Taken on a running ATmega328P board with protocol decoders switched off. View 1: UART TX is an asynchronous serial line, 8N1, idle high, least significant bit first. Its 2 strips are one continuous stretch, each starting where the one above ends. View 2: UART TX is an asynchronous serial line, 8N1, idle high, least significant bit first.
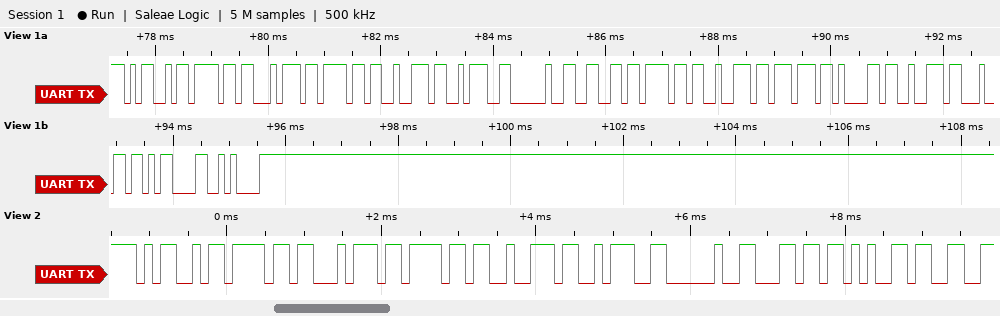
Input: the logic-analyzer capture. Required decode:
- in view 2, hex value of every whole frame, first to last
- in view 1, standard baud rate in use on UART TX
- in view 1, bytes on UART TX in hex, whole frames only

0x4D 0x6F 0x74 0x6F 0x72 0x3A 0x20 0x6C 0x65
9600 baud
0x4D 0x6F 0x74 0x6F 0x72 0x3A 0x20 0x66 0x6F 0x72 0x77 0x61 0x72 0x64 0x0D 0x0A
